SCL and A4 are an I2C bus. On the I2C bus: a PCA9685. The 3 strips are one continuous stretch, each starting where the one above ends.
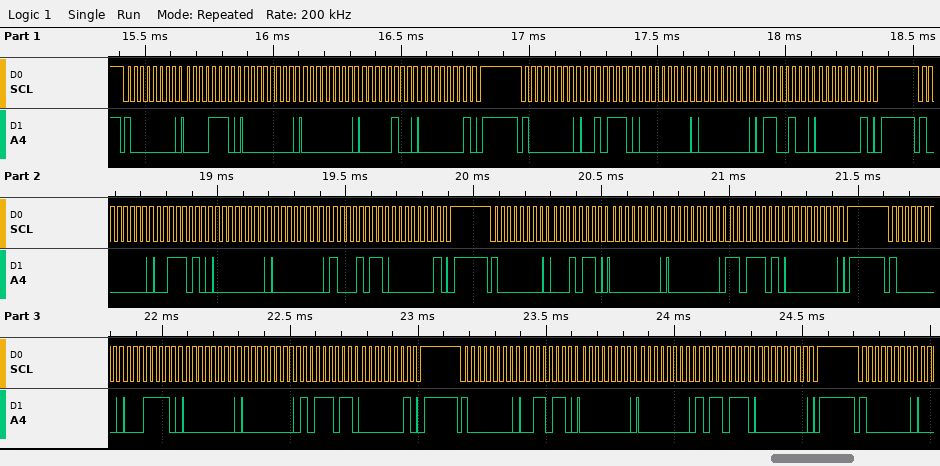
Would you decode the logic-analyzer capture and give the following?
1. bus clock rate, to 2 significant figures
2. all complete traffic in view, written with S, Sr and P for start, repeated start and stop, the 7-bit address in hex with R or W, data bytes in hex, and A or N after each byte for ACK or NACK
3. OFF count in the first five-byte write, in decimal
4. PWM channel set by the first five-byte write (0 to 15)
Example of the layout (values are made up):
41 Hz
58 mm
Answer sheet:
40 kHz
S 40W A 0E A 00 A 00 A 04 A 01 A P S 40W A 2E A 00 A 00 A 64 A 01 A P S 40W A 3A A 00 A 00 A 8B A 01 A P S 40W A 16 A 00 A 00 A DD A 00 A P S 40W A 1E A 00 A 00 A BB A 01 A P S 40W A 36 A 00 A 00 A B7 A 00 A P S 40W A
260
2
